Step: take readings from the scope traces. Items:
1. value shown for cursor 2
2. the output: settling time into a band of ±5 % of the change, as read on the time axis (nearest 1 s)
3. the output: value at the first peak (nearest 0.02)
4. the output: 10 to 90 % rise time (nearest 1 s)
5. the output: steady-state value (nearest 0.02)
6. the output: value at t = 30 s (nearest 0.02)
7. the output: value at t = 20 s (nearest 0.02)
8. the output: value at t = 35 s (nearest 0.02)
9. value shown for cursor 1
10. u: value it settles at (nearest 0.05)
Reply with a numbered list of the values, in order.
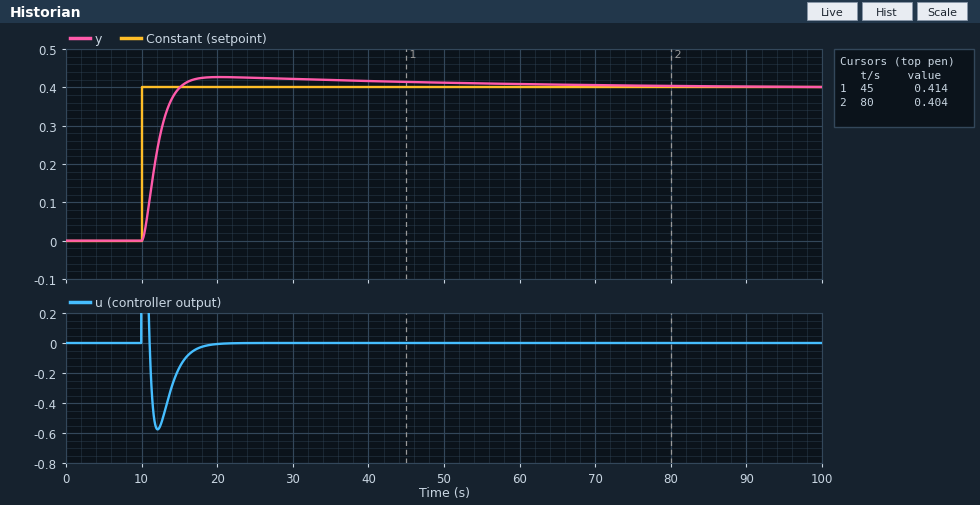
1. 0.404
2. 33 s
3. 0.42
4. 3 s
5. 0.40
6. 0.42
7. 0.42
8. 0.42
9. 0.414
10. 0.00
